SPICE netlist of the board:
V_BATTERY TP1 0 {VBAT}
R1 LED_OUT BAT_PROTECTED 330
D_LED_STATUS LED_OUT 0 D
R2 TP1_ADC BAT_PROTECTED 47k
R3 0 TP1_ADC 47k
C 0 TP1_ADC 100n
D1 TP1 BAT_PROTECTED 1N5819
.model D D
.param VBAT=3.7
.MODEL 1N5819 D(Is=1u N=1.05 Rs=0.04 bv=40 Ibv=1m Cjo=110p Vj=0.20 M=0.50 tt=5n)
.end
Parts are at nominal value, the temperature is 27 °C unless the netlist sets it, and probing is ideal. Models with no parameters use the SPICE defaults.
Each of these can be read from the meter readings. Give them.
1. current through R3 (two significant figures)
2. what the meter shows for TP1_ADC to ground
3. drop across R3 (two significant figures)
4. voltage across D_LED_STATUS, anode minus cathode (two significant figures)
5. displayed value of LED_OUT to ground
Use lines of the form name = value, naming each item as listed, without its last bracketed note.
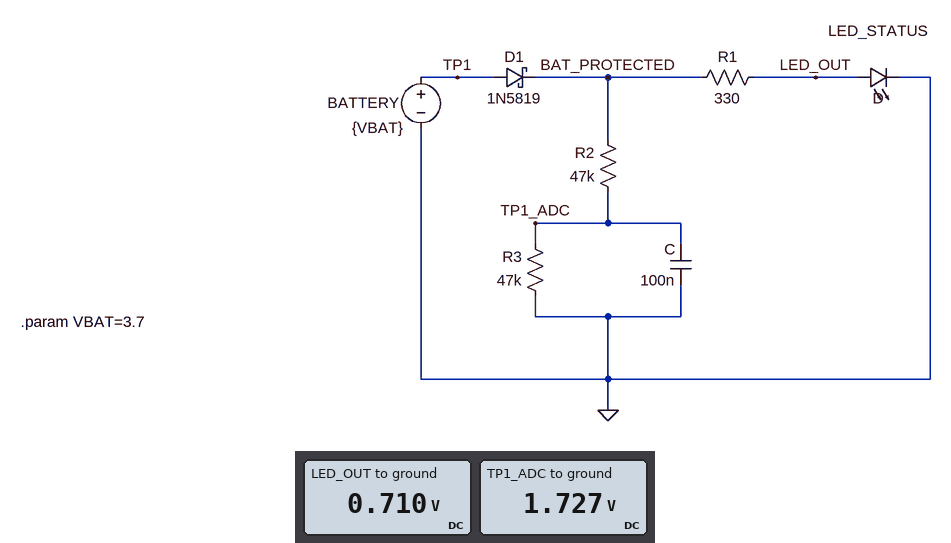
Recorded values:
current through R3 = 37 µA
what the meter shows for TP1_ADC to ground = 1.727 V
drop across R3 = 1.7 V
voltage across D_LED_STATUS, anode minus cathode = 710 mV
displayed value of LED_OUT to ground = 0.710 V
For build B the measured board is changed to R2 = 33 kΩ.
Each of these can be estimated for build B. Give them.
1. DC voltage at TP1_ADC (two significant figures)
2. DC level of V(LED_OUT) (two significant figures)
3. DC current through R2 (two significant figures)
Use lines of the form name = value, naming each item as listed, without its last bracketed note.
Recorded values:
DC voltage at TP1_ADC = 2.0 V
DC level of V(LED_OUT) = 710 mV
DC current through R2 = 43 µA
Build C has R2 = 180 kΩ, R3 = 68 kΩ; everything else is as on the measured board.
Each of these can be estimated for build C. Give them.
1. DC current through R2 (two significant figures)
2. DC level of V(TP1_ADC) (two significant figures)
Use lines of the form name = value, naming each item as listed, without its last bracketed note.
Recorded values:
DC current through R2 = 14 µA
DC level of V(TP1_ADC) = 950 mV
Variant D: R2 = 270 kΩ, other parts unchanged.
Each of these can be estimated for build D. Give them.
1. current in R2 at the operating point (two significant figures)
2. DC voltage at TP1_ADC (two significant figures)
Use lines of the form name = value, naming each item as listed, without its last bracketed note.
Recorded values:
current in R2 at the operating point = 11 µA
DC voltage at TP1_ADC = 510 mV
